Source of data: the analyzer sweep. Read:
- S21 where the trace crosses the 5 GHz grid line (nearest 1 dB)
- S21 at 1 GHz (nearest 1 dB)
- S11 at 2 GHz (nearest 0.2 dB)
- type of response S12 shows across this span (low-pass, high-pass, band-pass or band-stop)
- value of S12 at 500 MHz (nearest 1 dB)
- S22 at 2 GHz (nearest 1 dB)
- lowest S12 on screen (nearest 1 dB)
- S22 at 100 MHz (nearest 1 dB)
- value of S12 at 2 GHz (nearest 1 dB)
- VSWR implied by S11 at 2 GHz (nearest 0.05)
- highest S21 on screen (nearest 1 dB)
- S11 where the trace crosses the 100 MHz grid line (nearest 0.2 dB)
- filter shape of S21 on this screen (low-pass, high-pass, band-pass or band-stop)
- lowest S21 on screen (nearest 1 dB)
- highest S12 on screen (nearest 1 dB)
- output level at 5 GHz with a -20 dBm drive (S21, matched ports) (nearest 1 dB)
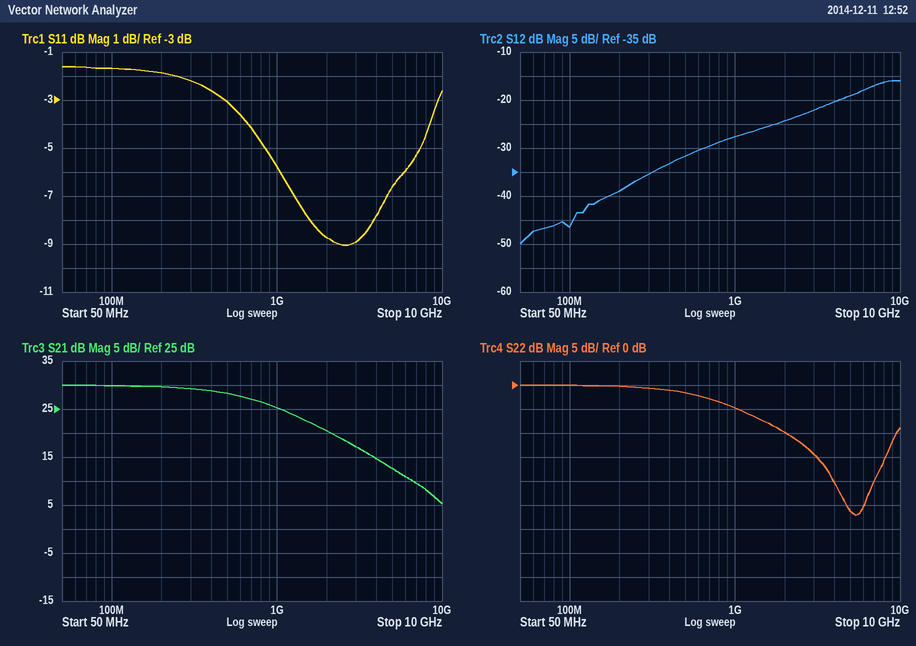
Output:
13 dB
25 dB
-8.8 dB
high-pass
-32 dB
-10 dB
-50 dB
0 dB
-24 dB
2.15
30 dB
-1.6 dB
low-pass
5 dB
-16 dB
-7 dBm
